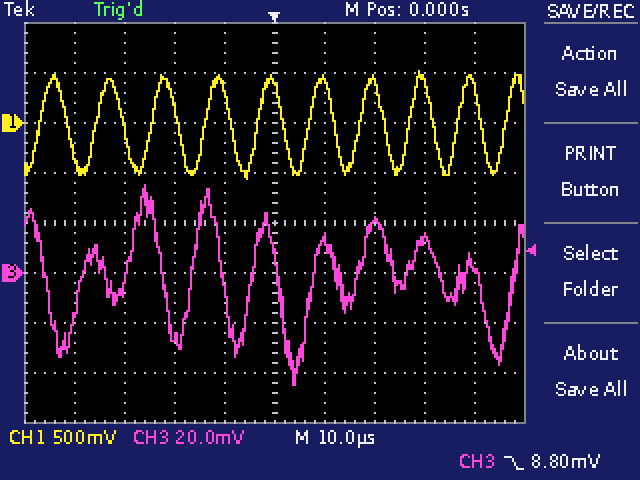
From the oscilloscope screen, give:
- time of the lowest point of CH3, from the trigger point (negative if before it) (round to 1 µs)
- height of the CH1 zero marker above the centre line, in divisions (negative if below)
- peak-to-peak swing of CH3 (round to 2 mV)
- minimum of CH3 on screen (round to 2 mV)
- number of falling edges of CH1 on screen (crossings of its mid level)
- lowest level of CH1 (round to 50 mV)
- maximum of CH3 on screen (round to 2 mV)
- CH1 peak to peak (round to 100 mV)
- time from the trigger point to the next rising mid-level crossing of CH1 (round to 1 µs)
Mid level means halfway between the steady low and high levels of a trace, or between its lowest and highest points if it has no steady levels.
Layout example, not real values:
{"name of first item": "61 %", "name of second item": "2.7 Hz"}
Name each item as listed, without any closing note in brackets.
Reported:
{"time of the lowest point of CH3, from the trigger point (negative if before it)": "+4 µs", "height of the CH1 zero marker above the centre line, in divisions": "+2.0 div", "peak-to-peak swing of CH3": "80 mV", "minimum of CH3 on screen": "-44 mV", "number of falling edges of CH1 on screen": "9", "lowest level of CH1": "-550 mV", "maximum of CH3 on screen": "36 mV", "CH1 peak to peak": "1.10 V", "time from the trigger point to the next rising mid-level crossing of CH1": "7 µs"}
